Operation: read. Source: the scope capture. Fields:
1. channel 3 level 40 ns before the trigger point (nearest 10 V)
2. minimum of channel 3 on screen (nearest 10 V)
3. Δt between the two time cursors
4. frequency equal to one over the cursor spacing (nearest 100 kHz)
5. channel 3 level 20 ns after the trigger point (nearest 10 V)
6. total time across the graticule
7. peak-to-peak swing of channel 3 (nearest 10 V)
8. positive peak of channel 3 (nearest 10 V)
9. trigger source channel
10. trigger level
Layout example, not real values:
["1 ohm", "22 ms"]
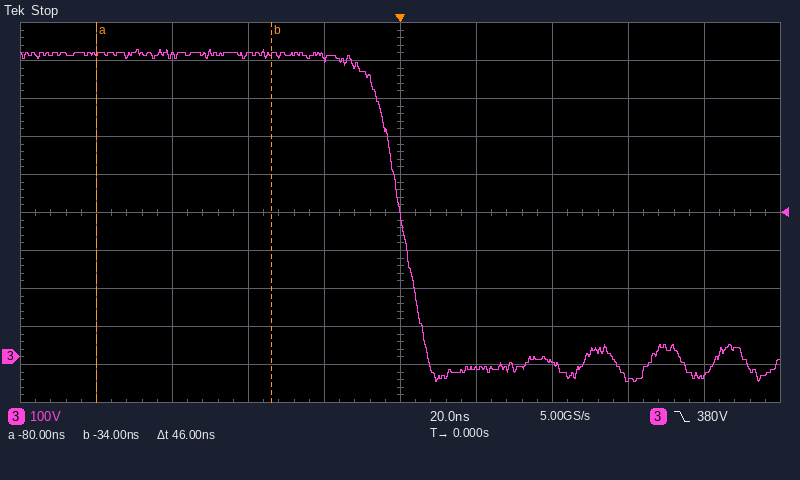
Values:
["790 V", "-60 V", "46 ns", "21.7 MHz", "-30 V", "200 ns", "870 V", "810 V", "channel 3", "380 V"]
